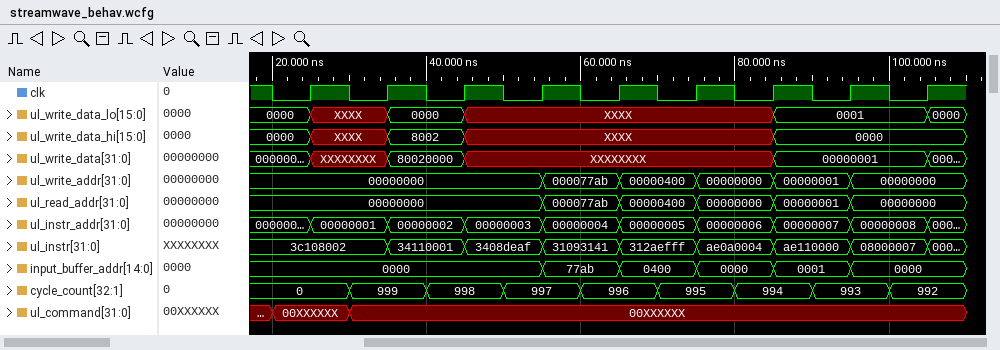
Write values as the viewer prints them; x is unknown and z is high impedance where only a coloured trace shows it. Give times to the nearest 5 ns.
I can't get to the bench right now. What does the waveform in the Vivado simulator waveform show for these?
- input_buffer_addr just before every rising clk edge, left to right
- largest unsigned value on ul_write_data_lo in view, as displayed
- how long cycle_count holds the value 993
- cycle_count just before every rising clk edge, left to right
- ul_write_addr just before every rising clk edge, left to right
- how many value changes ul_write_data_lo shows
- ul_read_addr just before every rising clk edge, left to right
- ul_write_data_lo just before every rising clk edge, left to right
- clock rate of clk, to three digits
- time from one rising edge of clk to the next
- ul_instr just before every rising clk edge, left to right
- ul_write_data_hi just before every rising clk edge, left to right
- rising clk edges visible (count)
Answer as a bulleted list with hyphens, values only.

- 0000, 0000, 0000, 0000, 77ab, 0400, 0000, 0001, 0000
- 0001
- 10 ns
- 0, 999, 998, 997, 996, 995, 994, 993, 992
- 00000000, 00000000, 00000000, 00000000, 000077ab, 00000400, 00000000, 00000001, 00000000
- 5
- 00000000, 00000000, 00000000, 00000000, 000077ab, 00000400, 00000000, 00000001, 00000000
- 0000, XXXX, 0000, XXXX, XXXX, XXXX, XXXX, 0001, 0001
- 100 MHz
- 10 ns
- 3c108002, 3c108002, 34110001, 3408deaf, 31093141, 312aefff, ae0a0004, ae110000, 08000007
- 0000, XXXX, 8002, XXXX, XXXX, XXXX, XXXX, 0000, 0000
- 9
